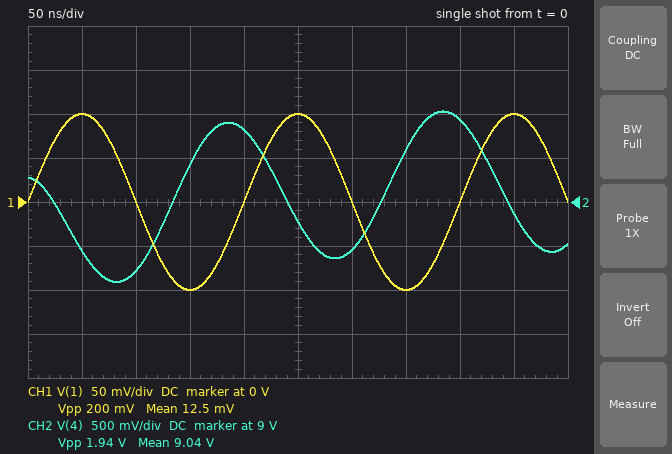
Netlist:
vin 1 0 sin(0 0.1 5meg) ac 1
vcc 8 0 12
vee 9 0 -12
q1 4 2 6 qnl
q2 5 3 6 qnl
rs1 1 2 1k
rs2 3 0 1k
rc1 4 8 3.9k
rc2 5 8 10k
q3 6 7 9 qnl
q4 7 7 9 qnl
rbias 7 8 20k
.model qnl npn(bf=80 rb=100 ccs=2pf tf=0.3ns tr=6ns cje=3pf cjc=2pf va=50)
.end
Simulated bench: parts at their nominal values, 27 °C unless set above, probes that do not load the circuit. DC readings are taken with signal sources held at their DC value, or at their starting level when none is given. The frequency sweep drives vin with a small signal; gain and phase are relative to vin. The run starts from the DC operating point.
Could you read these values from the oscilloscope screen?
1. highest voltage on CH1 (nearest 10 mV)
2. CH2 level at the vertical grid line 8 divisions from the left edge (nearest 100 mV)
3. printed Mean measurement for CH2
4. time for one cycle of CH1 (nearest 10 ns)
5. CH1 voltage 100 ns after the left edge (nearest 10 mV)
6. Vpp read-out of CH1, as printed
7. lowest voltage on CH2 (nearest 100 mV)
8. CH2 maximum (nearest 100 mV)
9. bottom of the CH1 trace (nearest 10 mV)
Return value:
100 mV
9.9 V
9.04 V
200 ns
0 V
200 mV
8.1 V
10.0 V
-100 mV
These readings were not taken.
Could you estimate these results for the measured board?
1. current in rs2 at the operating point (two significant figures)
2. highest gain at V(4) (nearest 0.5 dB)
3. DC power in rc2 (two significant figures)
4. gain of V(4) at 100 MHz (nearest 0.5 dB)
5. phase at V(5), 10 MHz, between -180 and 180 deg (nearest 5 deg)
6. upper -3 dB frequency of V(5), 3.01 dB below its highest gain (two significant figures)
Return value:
7.4 µA
31.0 dB
4.3 mW
-3.0 dB
-100 deg
950 kHz
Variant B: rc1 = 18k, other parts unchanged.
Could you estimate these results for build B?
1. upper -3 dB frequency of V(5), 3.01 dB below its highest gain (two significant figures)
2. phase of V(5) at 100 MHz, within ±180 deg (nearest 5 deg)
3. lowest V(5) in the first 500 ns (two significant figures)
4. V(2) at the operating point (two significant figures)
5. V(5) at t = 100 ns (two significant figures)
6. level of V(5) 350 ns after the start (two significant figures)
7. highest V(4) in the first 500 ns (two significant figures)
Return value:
370 kHz
-135 deg
4.1 V
-8.0 mV
5.9 V
4.8 V
1.1 V
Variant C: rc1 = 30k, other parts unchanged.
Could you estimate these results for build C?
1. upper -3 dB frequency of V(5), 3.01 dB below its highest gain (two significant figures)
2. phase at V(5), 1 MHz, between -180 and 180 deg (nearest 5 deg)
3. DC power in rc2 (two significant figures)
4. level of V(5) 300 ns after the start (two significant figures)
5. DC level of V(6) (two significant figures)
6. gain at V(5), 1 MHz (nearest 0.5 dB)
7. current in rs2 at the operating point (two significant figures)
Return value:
4.0 MHz
-15 deg
8.3 mW
3.3 V
-780 mV
18.0 dB
11 µA
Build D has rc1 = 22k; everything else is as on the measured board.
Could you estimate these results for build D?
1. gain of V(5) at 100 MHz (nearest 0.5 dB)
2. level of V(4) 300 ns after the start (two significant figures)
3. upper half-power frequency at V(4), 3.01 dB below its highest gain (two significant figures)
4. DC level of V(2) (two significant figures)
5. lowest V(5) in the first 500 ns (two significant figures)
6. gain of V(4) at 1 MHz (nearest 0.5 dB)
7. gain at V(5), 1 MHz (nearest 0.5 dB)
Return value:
-14.5 dB
-710 mV
4.7 MHz
-13 mV
3.3 V
10.5 dB
19.0 dB
